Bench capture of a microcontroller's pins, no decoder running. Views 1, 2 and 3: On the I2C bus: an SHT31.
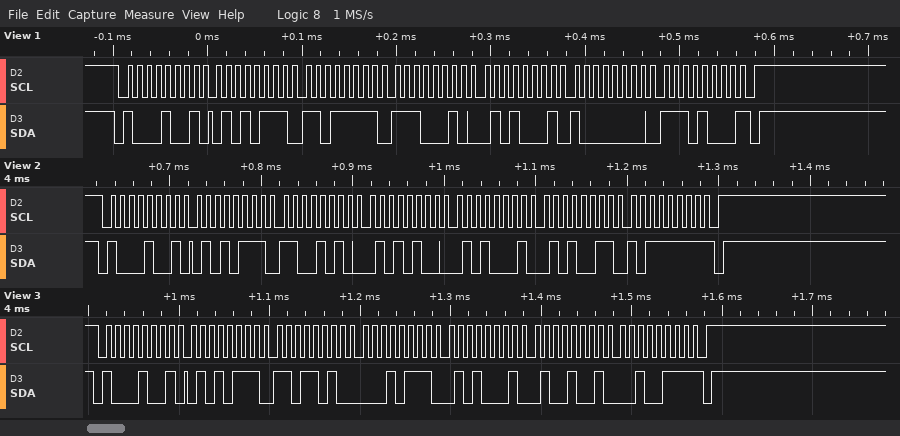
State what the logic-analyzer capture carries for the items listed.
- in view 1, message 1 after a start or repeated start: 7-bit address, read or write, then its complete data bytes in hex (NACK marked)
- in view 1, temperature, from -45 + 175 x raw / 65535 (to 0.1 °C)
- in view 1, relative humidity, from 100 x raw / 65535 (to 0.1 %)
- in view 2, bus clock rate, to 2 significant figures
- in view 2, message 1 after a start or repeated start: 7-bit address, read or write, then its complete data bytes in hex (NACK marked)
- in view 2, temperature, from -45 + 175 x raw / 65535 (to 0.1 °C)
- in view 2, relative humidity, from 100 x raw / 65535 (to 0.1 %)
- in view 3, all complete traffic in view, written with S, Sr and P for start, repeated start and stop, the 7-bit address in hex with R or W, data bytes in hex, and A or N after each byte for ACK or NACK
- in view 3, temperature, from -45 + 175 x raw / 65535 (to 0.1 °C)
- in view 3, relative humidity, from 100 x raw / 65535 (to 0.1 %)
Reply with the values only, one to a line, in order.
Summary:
0x44 read: 57 DF E2 51 80 E8 NACK
15.1 °C
31.8 %
100 kHz
0x44 read: 57 CA 54 51 53 BF NACK
15.0 °C
31.8 %
S 44R A 57 A DA A 17 A 51 A 49 A 27 N P
15.1 °C
31.8 %
